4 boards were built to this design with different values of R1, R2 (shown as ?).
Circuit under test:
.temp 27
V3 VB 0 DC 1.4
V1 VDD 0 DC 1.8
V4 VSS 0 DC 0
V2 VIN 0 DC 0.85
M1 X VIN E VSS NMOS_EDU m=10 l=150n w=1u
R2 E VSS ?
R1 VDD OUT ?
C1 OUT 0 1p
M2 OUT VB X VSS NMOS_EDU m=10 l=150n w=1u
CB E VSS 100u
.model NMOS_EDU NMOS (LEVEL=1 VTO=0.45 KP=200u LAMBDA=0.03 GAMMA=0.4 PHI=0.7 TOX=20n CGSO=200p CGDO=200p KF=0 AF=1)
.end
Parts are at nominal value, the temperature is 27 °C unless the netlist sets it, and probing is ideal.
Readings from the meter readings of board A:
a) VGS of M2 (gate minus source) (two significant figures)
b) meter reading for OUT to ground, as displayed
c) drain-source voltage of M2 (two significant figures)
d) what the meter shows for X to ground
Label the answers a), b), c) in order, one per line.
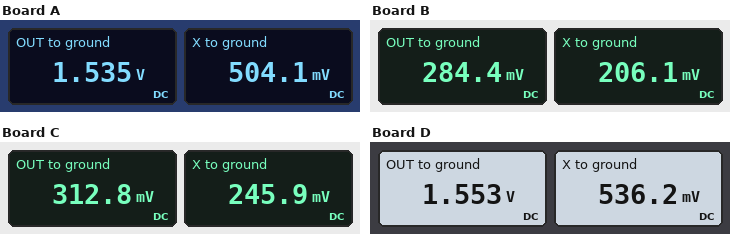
a) 900 mV
b) 1.535 V
c) 1.0 V
d) 504.1 mV
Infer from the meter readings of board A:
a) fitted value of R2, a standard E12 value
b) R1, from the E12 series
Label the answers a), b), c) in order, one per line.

a) 56 Ω
b) 330 Ω
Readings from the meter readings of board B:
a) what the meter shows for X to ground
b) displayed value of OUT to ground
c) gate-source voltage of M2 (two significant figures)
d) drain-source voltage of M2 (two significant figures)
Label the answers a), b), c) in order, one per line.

a) 206.1 mV
b) 284.4 mV
c) 1.2 V
d) 78 mV
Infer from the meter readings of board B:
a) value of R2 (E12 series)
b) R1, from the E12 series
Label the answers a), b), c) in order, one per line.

a) 33 Ω
b) 2.2 kΩ
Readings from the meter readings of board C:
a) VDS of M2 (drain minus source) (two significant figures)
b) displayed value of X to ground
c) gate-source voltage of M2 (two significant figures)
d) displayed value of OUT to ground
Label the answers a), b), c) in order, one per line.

a) 67 mV
b) 245.9 mV
c) 1.2 V
d) 312.8 mV
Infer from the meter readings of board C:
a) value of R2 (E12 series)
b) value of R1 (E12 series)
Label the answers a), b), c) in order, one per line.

a) 120 Ω
b) 2.7 kΩ
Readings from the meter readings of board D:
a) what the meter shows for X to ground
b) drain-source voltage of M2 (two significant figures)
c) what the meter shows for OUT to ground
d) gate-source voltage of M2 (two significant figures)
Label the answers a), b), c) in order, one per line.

a) 536.2 mV
b) 1.0 V
c) 1.553 V
d) 860 mV
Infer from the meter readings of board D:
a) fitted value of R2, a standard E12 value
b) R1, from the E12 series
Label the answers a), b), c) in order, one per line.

a) 120 Ω
b) 390 Ω
